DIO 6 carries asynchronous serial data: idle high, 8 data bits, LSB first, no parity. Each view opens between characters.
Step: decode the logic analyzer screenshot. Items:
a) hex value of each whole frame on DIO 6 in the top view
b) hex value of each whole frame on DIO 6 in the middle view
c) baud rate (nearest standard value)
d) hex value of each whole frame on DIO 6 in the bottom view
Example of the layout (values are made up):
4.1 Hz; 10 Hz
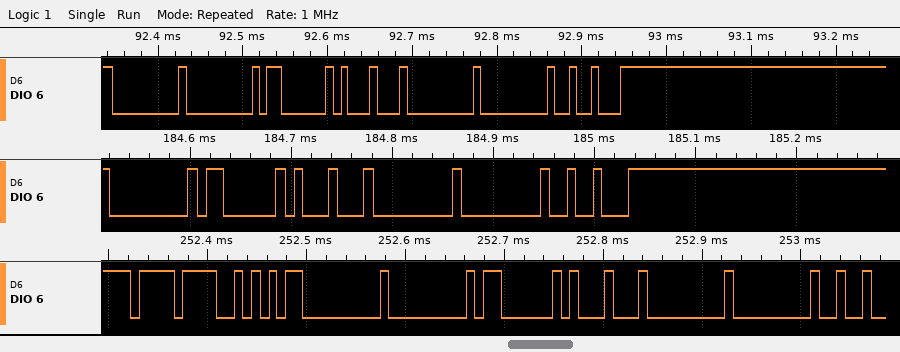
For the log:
00, 00, 03, 11, 00, 00, 12; 00, 03, 11, 00, 00, 12; 115200 baud; EF, AA, 00, 00, 03, 11, 00, 00
